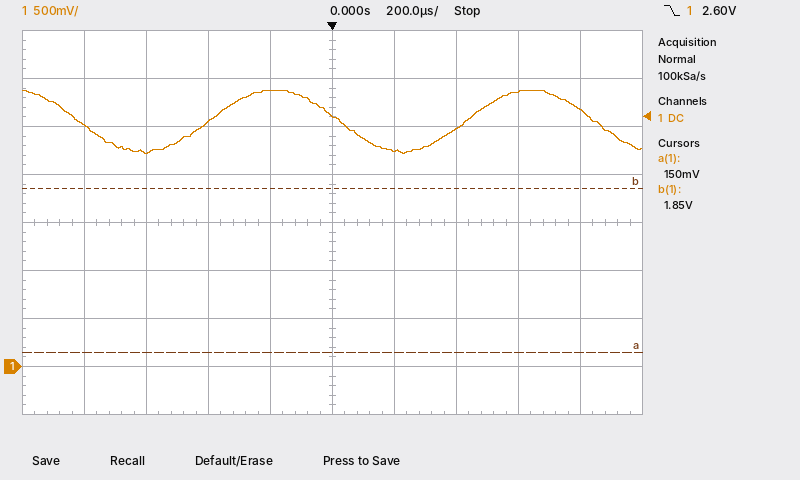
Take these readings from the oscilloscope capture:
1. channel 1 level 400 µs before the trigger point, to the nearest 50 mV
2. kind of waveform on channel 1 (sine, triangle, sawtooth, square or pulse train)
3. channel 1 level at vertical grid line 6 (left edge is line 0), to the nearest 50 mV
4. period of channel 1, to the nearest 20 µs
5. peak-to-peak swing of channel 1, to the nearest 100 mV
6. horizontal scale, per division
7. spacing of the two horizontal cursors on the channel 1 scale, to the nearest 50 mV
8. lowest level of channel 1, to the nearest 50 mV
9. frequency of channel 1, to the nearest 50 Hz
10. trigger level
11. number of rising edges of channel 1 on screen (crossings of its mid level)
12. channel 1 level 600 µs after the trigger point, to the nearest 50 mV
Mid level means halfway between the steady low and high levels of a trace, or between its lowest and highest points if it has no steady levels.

2.55 V
sine
2.25 V
840 µs
700 mV
200 µs
1.70 V
2.20 V
1.20 kHz
2.60 V
2
2.85 V
